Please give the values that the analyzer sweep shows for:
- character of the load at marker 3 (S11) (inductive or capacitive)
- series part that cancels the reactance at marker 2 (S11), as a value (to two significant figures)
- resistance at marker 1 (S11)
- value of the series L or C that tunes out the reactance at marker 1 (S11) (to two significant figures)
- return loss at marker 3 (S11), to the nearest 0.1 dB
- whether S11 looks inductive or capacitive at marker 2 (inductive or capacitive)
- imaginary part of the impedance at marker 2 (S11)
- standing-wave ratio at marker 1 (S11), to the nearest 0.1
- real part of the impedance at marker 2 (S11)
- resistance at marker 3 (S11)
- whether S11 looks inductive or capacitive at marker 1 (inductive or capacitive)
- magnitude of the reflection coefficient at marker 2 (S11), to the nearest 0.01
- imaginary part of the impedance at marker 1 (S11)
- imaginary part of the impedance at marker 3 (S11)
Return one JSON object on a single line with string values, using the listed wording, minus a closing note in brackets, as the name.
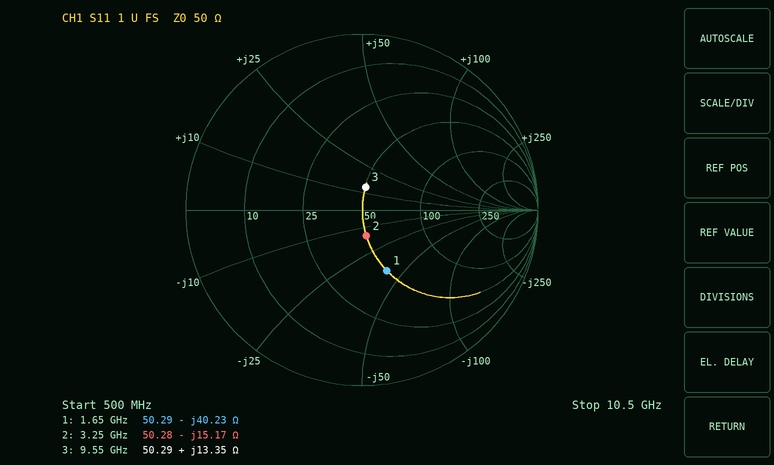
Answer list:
{"character of the load at marker 3 (S11)": "inductive", "series part that cancels the reactance at marker 2 (S11), as a value": "740 pH", "resistance at marker 1": "50.29 Ω", "value of the series L or C that tunes out the reactance at marker 1 (S11)": "3.9 nH", "return loss at marker 3 (S11), to the nearest 0.1 dB": "17.6 dB", "whether S11 looks inductive or capacitive at marker 2": "capacitive", "imaginary part of the impedance at marker 2": "-15.17 Ω", "standing-wave ratio at marker 1 (S11), to the nearest 0.1": "2.2", "real part of the impedance at marker 2": "50.28 Ω", "resistance at marker 3": "50.29 Ω", "whether S11 looks inductive or capacitive at marker 1": "capacitive", "magnitude of the reflection coefficient at marker 2 (S11), to the nearest 0.01": "0.15", "imaginary part of the impedance at marker 1": "-40.23 Ω", "imaginary part of the impedance at marker 3": "+13.35 Ω"}
